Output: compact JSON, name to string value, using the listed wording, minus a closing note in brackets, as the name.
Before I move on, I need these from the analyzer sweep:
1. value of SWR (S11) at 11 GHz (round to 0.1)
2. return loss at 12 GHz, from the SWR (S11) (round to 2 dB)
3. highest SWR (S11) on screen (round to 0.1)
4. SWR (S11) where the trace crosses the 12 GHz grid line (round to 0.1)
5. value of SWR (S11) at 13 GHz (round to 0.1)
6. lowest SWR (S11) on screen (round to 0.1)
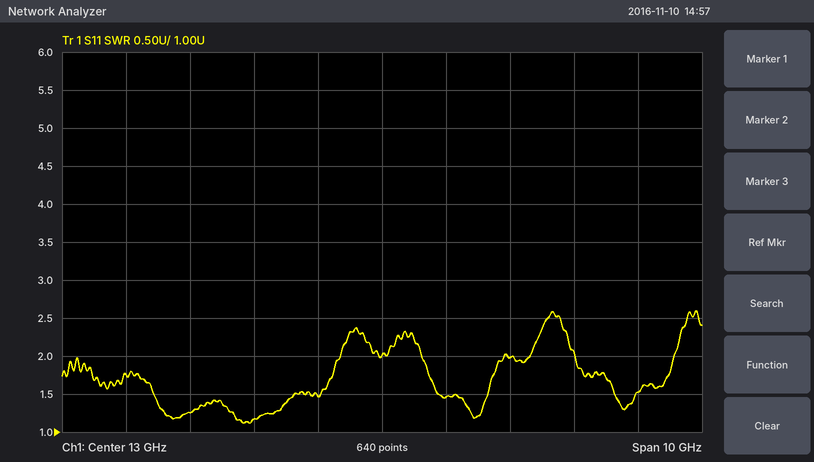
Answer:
{"value of SWR (S11) at 11 GHz": "1.2", "return loss at 12 GHz, from the SWR (S11)": "14 dB", "highest SWR (S11) on screen": "2.6", "SWR (S11) where the trace crosses the 12 GHz grid line": "1.5", "value of SWR (S11) at 13 GHz": "2.0", "lowest SWR (S11) on screen": "1.1"}
